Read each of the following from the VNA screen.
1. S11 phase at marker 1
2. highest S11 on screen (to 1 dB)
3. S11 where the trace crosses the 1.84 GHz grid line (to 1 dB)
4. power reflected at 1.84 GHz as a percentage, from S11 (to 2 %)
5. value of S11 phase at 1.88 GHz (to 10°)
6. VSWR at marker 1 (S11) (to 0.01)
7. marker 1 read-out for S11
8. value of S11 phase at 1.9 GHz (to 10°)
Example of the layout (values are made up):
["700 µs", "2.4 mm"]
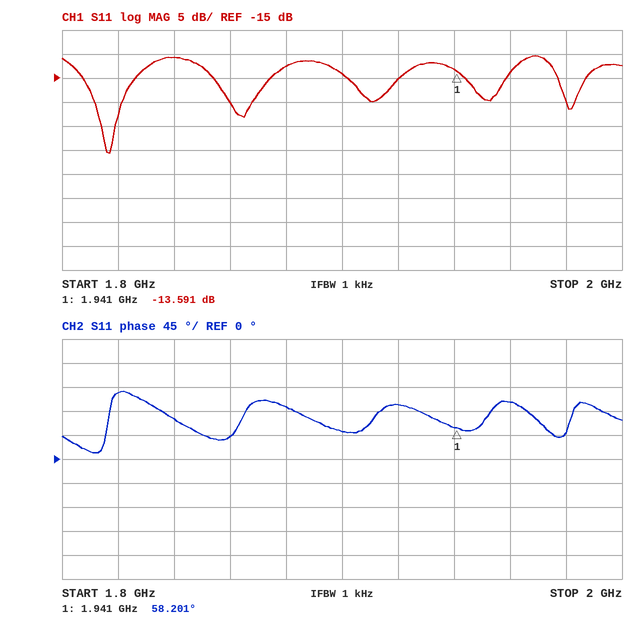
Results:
["58.201°", "-10 dB", "-11 dB", "8 %", "100°", "1.53", "-13.591 dB", "50°"]
